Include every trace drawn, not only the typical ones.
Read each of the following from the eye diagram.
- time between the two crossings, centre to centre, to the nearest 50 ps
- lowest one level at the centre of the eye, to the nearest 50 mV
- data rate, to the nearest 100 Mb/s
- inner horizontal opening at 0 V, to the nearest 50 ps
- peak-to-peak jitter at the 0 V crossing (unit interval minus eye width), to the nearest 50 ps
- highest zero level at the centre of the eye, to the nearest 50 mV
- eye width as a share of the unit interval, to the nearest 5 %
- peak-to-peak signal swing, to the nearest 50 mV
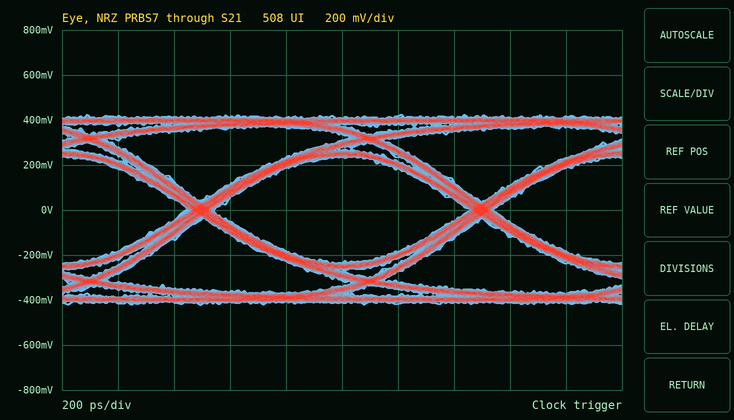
1.00 ns
250 mV
1.0 Gb/s
900 ps
100 ps
-250 mV
90 %
850 mV
